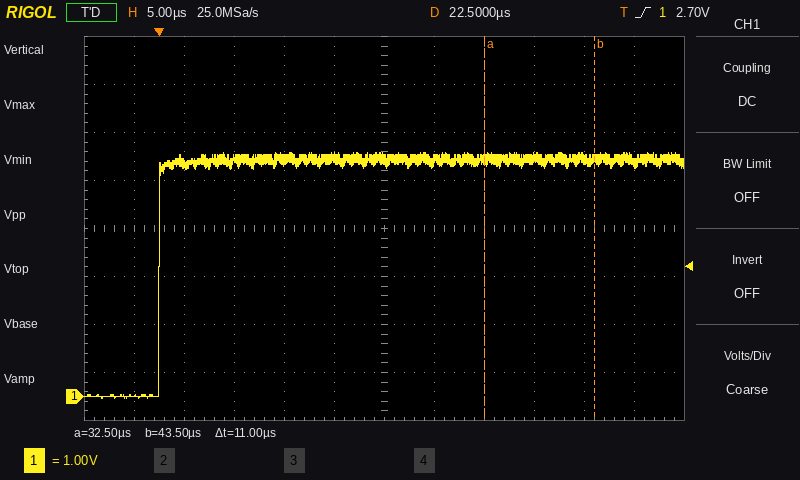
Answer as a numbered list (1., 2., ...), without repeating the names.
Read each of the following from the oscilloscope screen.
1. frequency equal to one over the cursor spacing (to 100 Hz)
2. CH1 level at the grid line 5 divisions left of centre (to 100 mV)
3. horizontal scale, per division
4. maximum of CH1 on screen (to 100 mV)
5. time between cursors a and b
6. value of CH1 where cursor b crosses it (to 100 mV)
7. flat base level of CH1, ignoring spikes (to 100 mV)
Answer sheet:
1. 90.9 kHz
2. 0.0 V
3. 5 µs
4. 5.1 V
5. 11 µs
6. 4.9 V
7. 0.0 V
